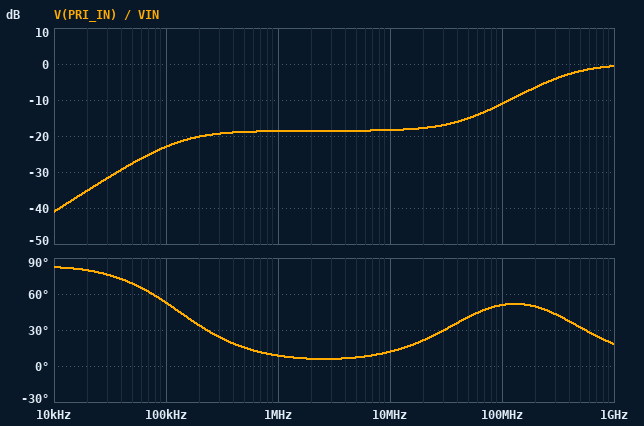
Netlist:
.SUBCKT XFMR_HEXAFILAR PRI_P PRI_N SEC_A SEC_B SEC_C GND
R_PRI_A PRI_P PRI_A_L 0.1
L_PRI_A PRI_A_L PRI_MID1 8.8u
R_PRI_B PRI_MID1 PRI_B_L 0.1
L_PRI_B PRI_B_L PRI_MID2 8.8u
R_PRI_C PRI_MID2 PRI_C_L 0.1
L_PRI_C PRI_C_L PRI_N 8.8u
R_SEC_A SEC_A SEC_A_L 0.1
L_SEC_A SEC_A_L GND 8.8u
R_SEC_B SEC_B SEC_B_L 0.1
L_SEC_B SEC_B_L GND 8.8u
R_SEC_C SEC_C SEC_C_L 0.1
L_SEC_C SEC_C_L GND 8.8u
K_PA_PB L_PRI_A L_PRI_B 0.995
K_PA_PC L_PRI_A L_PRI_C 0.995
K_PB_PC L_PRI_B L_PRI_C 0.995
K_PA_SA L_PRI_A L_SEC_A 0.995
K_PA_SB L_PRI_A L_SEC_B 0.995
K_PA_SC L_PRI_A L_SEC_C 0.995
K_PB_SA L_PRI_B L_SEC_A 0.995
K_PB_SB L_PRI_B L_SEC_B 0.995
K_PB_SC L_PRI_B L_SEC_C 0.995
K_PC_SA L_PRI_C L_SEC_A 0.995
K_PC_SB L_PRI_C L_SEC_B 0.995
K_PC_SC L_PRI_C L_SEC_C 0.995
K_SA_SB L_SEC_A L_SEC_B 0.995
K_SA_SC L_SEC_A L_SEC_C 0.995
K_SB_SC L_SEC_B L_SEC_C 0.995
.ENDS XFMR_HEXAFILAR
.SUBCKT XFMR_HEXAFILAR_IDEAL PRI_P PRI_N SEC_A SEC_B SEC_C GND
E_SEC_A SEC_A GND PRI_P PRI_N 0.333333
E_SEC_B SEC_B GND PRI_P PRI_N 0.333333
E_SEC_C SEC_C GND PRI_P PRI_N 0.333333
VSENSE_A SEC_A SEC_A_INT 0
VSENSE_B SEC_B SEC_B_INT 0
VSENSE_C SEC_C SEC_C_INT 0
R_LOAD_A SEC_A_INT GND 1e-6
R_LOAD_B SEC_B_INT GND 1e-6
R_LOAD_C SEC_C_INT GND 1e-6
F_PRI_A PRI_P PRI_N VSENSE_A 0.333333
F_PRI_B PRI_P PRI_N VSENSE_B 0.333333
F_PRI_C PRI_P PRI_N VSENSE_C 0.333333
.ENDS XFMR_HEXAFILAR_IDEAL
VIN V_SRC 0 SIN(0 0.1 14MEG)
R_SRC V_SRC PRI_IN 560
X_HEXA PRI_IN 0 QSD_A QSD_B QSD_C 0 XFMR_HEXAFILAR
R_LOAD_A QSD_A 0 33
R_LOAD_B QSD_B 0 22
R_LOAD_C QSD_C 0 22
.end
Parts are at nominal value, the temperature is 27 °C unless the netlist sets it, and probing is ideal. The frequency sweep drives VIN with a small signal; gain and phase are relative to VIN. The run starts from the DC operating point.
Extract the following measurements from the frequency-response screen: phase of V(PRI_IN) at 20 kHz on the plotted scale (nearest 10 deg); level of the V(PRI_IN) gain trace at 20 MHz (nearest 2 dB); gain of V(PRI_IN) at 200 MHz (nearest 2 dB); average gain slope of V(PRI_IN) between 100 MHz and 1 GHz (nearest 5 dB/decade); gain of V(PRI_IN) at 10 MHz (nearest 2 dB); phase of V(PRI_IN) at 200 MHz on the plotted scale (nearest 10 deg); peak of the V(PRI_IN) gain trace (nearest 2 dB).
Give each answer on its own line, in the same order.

80 deg
-18 dB
-6 dB
10 dB/decade
-18 dB
50 deg
0 dB
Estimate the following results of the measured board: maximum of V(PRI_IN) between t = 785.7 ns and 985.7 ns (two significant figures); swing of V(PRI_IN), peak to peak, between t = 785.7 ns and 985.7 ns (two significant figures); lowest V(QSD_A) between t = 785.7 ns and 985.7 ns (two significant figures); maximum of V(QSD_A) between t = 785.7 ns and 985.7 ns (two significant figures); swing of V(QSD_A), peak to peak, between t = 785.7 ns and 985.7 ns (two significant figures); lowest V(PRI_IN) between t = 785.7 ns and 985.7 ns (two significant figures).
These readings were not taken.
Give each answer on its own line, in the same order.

12 mV
25 mV
-3.9 mV
3.9 mV
7.8 mV
-12 mV
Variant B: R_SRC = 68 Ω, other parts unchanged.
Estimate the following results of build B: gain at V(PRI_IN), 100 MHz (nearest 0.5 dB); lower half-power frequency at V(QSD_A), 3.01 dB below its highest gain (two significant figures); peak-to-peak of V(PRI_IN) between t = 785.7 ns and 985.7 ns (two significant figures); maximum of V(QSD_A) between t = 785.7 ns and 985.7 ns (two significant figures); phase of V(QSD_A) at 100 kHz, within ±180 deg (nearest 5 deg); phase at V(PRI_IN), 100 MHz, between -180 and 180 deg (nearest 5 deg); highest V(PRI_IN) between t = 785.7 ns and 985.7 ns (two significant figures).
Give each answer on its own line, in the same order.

-1.5 dB
72 kHz
110 mV
17 mV
35 deg
15 deg
54 mV
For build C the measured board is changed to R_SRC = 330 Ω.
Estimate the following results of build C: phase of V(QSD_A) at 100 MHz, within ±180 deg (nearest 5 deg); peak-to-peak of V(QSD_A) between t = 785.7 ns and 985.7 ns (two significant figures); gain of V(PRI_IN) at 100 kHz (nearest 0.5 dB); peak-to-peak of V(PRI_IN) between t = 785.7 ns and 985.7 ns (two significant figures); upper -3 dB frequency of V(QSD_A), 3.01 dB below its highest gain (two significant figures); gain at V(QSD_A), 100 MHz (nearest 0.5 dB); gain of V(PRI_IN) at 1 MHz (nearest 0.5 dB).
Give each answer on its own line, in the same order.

-15 deg
12 mV
-18.5 dB
39 mV
340 MHz
-23.5 dB
-14.5 dB
